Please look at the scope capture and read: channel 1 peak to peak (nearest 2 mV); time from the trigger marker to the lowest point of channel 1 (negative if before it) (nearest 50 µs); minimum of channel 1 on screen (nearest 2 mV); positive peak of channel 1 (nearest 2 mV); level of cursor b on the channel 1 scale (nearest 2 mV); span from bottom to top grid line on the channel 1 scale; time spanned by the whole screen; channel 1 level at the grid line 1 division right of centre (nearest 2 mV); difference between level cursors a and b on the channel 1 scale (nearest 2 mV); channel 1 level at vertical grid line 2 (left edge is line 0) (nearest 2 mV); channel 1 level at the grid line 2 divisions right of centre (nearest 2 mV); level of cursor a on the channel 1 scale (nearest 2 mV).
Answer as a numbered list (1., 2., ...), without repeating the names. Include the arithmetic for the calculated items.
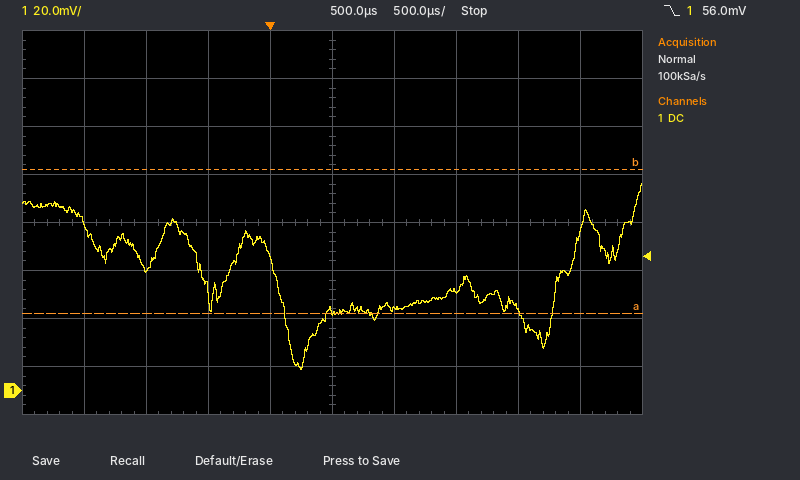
1. 86 mV − (8 mV) = 78 mV
2. +250 µs
3. 8 mV
4. 86 mV
5. 92 mV
6. 160 mV
7. 5 ms
8. 34 mV
9. 60 mV
10. 50 mV
11. 42 mV
12. 32 mV
